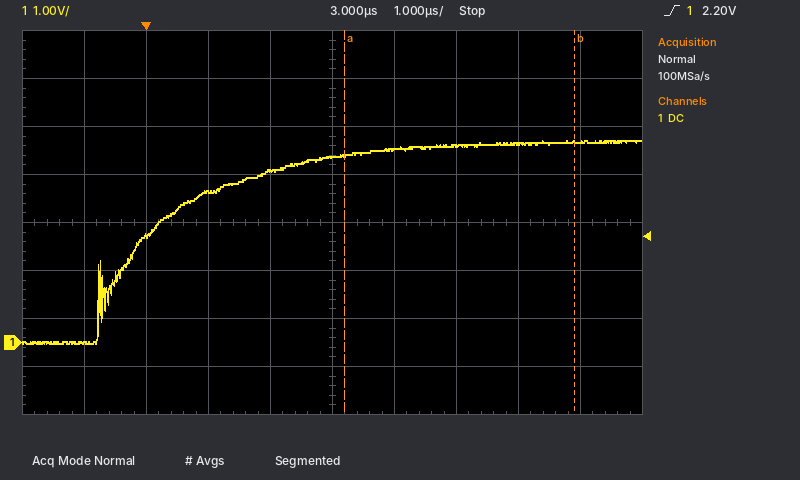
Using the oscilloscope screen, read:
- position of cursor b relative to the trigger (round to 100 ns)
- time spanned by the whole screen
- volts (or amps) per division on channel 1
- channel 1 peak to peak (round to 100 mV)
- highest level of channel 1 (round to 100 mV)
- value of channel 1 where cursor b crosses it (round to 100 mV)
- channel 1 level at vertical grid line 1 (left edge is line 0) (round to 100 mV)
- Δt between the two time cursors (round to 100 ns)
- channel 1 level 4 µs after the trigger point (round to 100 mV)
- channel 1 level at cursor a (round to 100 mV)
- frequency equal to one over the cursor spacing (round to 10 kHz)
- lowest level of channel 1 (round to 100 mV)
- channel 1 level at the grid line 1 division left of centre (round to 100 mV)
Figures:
+6.9 µs
10 µs
1 V
4.2 V
4.2 V
4.2 V
0.0 V
3.7 µs
4.0 V
3.9 V
270 kHz
0.0 V
3.6 V
